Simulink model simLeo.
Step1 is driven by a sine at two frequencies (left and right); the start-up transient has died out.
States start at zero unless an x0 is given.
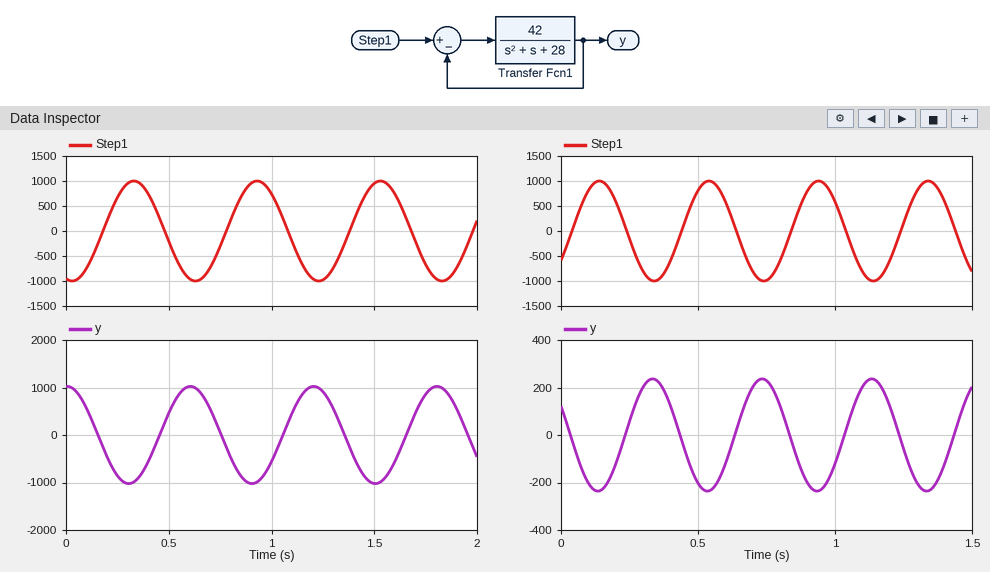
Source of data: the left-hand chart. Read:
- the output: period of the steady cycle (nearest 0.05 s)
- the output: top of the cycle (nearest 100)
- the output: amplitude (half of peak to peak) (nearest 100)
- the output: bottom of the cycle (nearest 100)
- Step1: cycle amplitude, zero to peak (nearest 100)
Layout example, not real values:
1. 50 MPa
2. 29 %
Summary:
1. 0.60 s
2. 1000
3. 1000
4. -1000
5. 1000
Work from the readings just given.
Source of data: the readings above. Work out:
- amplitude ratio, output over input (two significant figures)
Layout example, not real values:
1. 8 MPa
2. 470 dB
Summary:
1. 1.0
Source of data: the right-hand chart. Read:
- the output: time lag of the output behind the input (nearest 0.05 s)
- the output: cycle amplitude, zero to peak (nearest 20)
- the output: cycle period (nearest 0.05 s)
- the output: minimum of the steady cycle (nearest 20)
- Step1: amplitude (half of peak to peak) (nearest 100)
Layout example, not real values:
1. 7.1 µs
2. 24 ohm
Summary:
1. 0.20 s
2. 240
3. 0.40 s
4. -240
5. 1000
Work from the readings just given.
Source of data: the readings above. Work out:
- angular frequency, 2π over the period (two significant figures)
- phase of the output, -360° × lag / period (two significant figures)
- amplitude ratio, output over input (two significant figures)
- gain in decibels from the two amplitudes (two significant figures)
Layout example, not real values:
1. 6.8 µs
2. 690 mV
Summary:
1. 16 rad/s
2. -180°
3. 0.24
4. -12 dB
